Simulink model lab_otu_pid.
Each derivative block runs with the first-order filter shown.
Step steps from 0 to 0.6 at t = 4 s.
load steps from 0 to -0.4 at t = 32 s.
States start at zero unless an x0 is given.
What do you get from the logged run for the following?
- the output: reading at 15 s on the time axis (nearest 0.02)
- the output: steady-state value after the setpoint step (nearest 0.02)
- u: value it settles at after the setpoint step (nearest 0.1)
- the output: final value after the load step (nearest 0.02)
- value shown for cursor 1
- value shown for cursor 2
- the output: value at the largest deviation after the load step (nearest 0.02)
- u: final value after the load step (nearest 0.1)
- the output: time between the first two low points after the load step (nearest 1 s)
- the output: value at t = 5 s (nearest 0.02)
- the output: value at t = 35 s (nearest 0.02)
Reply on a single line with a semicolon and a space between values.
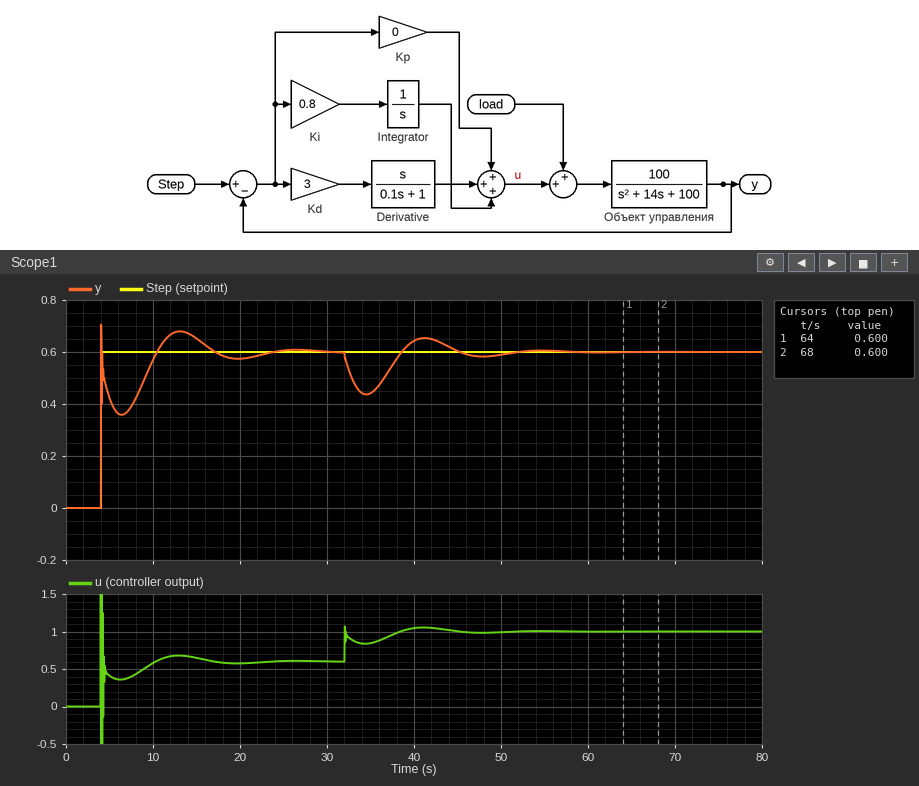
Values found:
0.66; 0.60; 0.6; 0.60; 0.600; 0.600; 0.44; 1.0; 13 s; 0.42; 0.44
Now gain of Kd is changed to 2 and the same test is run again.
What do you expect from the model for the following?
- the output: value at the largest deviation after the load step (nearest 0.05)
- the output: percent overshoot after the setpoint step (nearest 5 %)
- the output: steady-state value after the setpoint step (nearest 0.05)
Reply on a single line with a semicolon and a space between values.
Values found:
0.40; 20 %; 0.60
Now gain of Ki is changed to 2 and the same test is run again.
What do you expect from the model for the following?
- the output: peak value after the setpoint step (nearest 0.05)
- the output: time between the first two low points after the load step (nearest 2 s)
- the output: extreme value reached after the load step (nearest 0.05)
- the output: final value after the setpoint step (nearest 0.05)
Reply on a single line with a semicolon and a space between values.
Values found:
0.70; 8 s; 0.50; 0.60
